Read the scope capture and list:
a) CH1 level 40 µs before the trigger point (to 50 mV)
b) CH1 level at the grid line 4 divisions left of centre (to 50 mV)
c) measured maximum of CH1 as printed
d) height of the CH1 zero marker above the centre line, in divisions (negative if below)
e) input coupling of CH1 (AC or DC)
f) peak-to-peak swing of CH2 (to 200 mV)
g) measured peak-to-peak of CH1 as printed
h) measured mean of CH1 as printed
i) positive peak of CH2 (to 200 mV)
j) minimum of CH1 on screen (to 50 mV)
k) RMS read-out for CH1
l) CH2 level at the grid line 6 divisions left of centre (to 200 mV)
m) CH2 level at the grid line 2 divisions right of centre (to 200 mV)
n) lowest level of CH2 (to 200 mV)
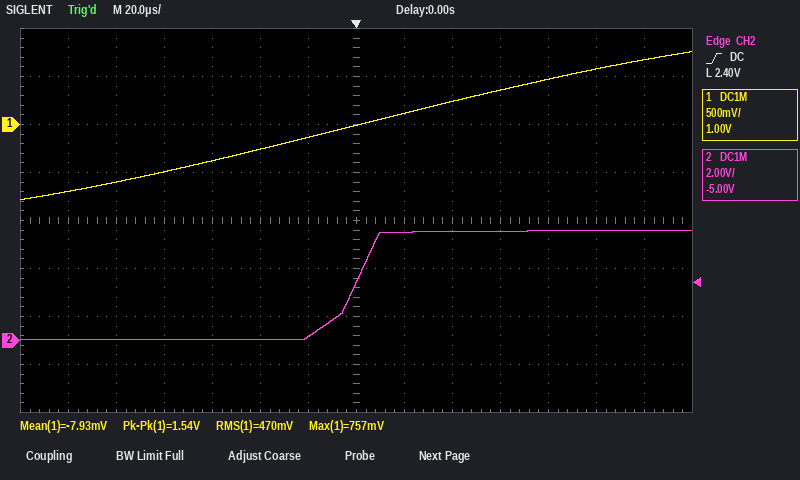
-250 mV
-500 mV
757 mV
+2.0 div
DC
4.6 V
1.54 V
-7.93 mV
4.6 V
-800 mV
470 mV
0.0 V
4.6 V
0.0 V
